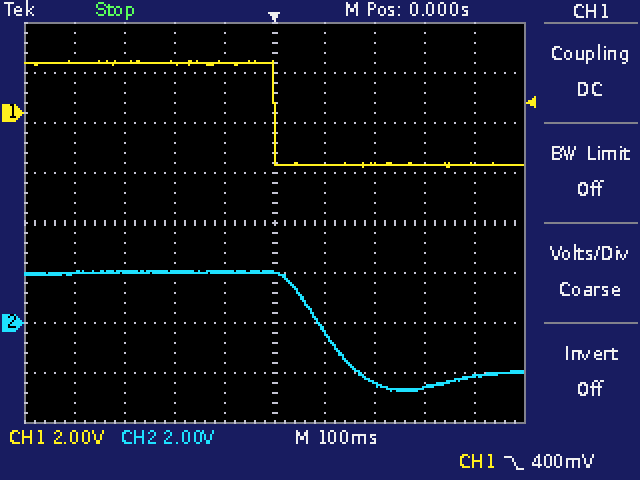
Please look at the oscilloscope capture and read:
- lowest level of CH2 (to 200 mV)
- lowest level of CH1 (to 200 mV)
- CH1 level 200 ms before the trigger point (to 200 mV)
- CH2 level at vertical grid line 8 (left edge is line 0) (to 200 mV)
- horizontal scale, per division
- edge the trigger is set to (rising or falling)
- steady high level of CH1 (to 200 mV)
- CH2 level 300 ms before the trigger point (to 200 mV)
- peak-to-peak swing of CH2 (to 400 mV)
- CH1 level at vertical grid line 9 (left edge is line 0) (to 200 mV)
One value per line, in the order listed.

-2.8 V
-2.2 V
2.0 V
-2.6 V
100 ms
falling
2.0 V
2.0 V
4.8 V
-2.0 V
